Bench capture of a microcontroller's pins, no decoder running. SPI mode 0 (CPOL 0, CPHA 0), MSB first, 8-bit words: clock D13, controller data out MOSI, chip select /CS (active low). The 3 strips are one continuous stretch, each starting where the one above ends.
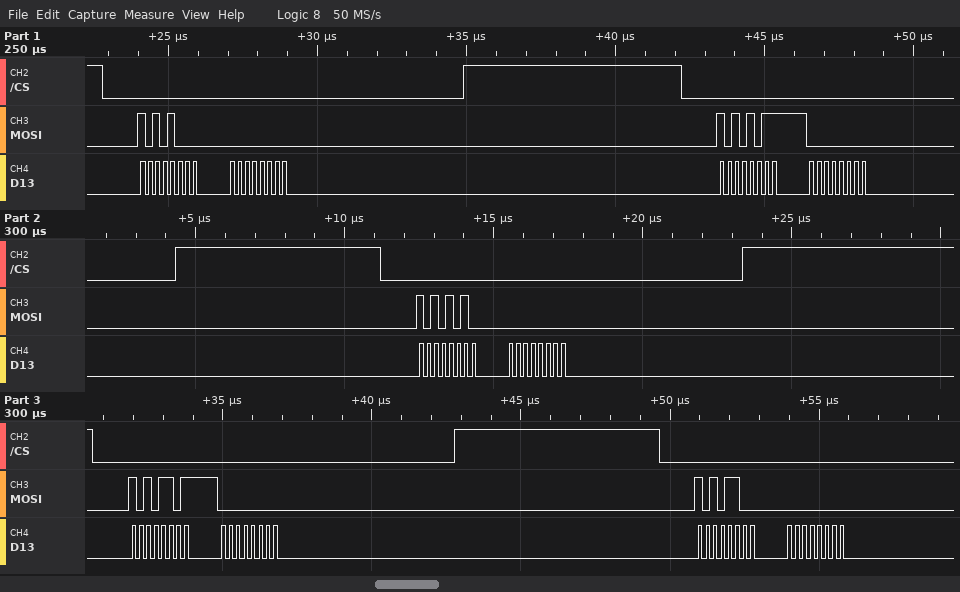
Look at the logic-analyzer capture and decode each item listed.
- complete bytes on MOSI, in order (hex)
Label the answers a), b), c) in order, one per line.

a) A8 00 AB 00 AA 00 AD 00 AC 00
